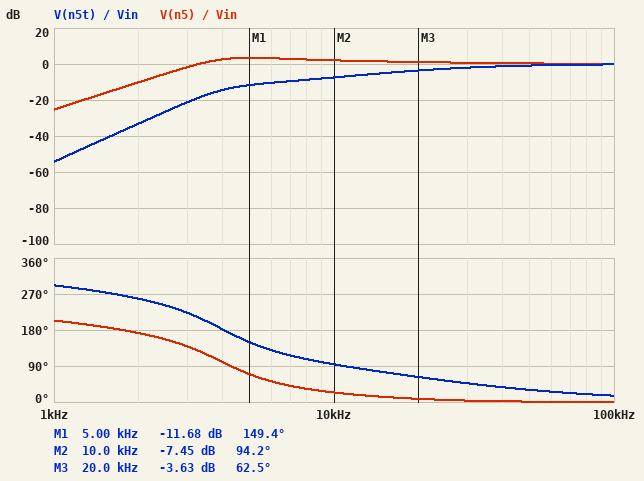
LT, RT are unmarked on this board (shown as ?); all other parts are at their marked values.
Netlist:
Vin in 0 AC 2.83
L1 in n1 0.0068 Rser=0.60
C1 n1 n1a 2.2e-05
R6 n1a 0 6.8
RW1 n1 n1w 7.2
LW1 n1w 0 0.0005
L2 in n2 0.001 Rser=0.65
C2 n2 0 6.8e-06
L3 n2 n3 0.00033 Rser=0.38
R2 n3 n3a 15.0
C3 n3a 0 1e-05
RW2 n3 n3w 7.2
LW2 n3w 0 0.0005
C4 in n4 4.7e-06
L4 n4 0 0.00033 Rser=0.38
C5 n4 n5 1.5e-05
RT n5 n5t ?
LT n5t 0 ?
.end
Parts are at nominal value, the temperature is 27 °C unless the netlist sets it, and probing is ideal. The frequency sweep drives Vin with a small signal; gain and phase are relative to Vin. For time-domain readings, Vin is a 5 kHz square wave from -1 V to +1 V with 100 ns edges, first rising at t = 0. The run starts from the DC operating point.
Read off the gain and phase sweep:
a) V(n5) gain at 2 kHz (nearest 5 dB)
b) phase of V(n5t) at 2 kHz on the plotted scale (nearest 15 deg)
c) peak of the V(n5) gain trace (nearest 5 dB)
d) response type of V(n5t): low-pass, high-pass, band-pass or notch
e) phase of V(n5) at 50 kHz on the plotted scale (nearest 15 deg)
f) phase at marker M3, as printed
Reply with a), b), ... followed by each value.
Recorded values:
a) -10 dB
b) 255 deg
c) 5 dB
d) high-pass
e) 0 deg
f) 62.5 deg
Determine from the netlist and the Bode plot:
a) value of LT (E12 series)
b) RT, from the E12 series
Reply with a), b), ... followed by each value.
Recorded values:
a) 68 µH
b) 12 Ω
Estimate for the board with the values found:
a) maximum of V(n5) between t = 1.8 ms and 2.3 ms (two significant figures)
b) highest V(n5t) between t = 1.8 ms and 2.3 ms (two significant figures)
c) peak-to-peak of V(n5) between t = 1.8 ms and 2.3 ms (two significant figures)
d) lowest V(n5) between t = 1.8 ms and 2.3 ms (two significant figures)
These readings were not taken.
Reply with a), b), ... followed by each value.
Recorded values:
a) 2.9 V
b) 2.0 V
c) 5.9 V
d) -2.9 V
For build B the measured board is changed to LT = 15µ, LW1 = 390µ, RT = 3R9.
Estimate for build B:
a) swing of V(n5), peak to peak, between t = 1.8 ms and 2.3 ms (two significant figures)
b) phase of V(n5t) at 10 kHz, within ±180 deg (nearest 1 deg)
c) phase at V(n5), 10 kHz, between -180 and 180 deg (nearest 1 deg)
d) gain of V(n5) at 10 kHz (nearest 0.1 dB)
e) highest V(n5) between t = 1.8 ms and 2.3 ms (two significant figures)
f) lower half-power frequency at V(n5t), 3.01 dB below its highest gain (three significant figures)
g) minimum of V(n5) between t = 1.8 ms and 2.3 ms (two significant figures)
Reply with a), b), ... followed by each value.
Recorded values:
a) 4.4 V
b) 137 deg
c) 61 deg
d) -1.5 dB
e) 2.2 V
f) 30.6 kHz
g) -2.2 V
